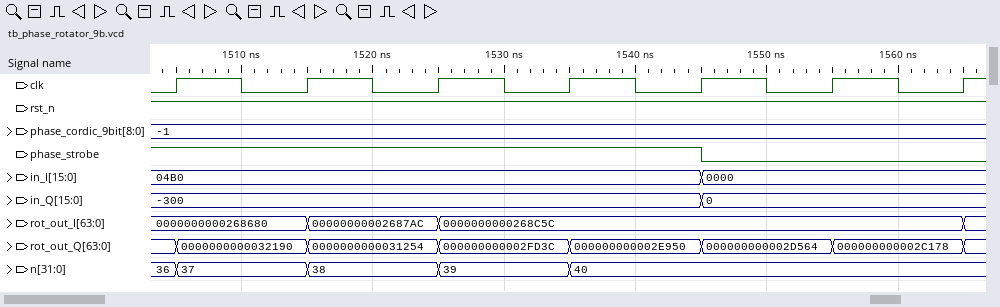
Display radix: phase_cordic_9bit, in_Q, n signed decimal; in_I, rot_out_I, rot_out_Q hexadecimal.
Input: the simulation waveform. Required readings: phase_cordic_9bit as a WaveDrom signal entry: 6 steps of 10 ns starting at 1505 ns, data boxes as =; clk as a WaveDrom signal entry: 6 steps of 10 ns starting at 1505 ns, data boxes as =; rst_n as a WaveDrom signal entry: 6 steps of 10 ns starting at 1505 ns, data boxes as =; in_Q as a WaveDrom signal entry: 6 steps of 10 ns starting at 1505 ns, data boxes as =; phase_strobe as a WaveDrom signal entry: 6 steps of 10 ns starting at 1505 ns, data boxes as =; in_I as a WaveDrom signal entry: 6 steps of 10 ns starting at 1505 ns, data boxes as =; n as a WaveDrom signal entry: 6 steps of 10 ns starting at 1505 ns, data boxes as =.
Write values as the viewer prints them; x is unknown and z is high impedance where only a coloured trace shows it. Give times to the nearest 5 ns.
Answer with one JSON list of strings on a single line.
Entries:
["{name: 'phase_cordic_9bit', wave: '=.....', data: '-1'}", "{name: 'clk', wave: 'p.....'}", "{name: 'rst_n', wave: '1.....'}", "{name: 'in_Q', wave: '=...=.', data: '-300 0'}", "{name: 'phase_strobe', wave: '1...0.'}", "{name: 'in_I', wave: '=...=.', data: '04B0 0000'}", "{name: 'n', wave: '====..', data: '37 38 39 40'}"]
